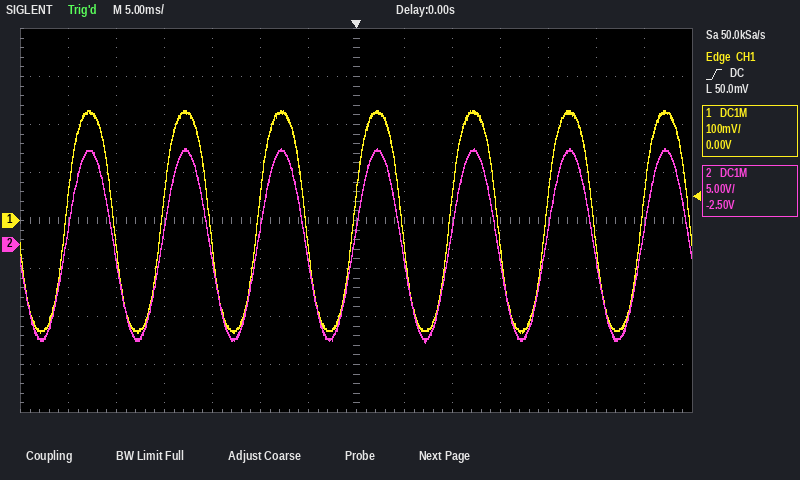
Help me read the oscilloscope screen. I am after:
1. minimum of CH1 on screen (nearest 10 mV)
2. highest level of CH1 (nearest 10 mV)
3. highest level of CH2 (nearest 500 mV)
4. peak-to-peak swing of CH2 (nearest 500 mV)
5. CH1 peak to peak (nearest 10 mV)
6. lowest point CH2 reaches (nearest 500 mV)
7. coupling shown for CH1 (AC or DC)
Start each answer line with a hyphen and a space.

- -230 mV
- 230 mV
- 10.0 V
- 20.0 V
- 460 mV
- -10.0 V
- DC
